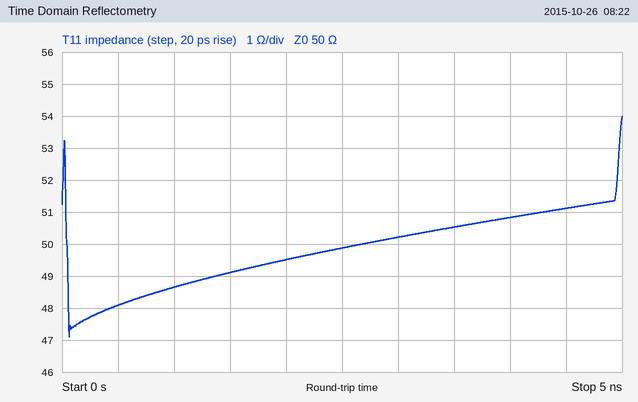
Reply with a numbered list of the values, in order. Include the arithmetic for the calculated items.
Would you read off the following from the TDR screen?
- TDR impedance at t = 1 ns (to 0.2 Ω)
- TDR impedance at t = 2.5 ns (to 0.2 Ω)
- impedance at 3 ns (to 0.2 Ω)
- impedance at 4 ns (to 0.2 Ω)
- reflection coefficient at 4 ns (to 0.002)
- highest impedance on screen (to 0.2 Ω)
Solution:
1. 48.6 Ω
2. 49.8 Ω
3. 50.2 Ω
4. 50.8 Ω
5. (50.8 − 50)/(50.8 + 50) ≈ +0.008
6. 54.0 Ω
